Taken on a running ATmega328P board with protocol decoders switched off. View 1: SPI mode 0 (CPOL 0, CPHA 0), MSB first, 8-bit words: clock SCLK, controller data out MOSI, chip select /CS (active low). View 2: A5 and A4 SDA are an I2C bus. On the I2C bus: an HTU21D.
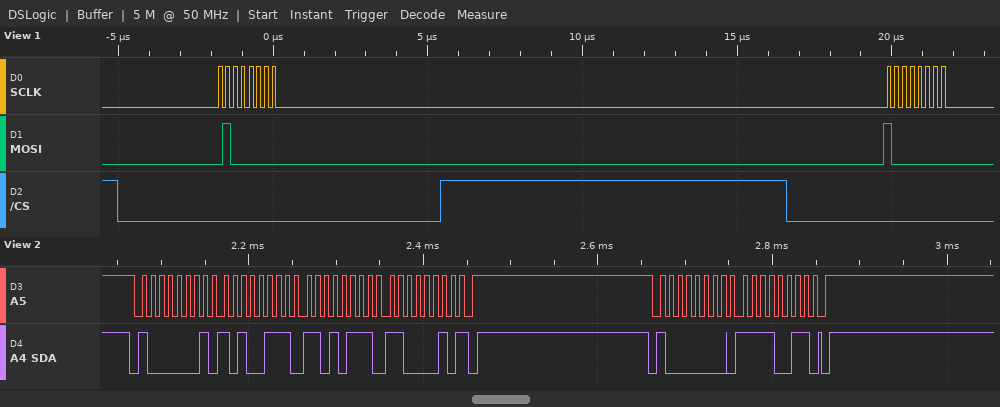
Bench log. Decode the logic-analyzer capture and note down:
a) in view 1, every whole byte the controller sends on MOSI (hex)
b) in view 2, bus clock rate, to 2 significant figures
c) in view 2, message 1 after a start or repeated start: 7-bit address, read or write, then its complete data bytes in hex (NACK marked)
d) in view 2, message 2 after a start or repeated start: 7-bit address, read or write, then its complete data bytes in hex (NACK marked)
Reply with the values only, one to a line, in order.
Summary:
40 80
100 kHz
0x40 read: A7 D7 C2 NACK
0x40 write: F3
